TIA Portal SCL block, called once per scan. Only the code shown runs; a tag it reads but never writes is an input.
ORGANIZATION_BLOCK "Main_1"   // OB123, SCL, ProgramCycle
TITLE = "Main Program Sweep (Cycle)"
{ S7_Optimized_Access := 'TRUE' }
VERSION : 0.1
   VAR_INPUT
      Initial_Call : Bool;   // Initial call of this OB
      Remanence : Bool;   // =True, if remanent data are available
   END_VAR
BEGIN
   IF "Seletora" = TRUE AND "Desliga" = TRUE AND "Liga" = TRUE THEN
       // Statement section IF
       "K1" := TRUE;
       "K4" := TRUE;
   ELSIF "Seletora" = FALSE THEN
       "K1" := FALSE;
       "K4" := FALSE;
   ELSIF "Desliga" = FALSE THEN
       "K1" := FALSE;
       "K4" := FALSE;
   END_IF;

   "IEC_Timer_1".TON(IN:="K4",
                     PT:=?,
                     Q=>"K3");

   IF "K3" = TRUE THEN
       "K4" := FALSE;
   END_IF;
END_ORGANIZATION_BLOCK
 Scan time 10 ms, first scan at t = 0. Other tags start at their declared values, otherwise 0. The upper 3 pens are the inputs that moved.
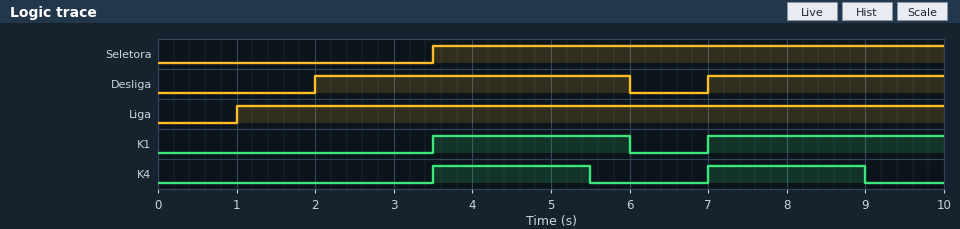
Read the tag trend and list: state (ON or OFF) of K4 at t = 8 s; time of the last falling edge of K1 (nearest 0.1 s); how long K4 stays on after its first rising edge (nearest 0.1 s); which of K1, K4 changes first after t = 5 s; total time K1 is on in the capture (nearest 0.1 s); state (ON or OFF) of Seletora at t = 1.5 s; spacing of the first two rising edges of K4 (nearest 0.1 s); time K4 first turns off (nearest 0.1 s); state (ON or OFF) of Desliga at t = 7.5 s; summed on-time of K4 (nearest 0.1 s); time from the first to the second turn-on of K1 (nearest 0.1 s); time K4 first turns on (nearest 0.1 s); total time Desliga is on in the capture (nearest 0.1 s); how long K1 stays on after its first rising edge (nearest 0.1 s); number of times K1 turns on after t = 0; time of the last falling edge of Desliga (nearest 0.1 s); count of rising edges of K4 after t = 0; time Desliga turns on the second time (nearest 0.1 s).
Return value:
ON
6.0 s
2.0 s
K4
5.5 s
OFF
3.5 s
5.5 s
ON
4.0 s
3.5 s
3.5 s
7.0 s
2.5 s
2
6.0 s
2
7.0 s
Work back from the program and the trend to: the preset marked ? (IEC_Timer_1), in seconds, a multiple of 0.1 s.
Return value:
2.0 s
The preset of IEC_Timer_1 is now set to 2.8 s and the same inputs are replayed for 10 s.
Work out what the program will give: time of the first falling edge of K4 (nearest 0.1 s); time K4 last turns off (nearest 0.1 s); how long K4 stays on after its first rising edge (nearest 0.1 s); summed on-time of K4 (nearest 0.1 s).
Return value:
6.0 s
9.8 s
2.5 s
5.3 s
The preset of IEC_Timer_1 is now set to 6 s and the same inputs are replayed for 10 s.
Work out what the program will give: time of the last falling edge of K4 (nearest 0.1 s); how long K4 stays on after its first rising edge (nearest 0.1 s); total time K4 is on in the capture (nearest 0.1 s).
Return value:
6.0 s
2.5 s
5.5 s
